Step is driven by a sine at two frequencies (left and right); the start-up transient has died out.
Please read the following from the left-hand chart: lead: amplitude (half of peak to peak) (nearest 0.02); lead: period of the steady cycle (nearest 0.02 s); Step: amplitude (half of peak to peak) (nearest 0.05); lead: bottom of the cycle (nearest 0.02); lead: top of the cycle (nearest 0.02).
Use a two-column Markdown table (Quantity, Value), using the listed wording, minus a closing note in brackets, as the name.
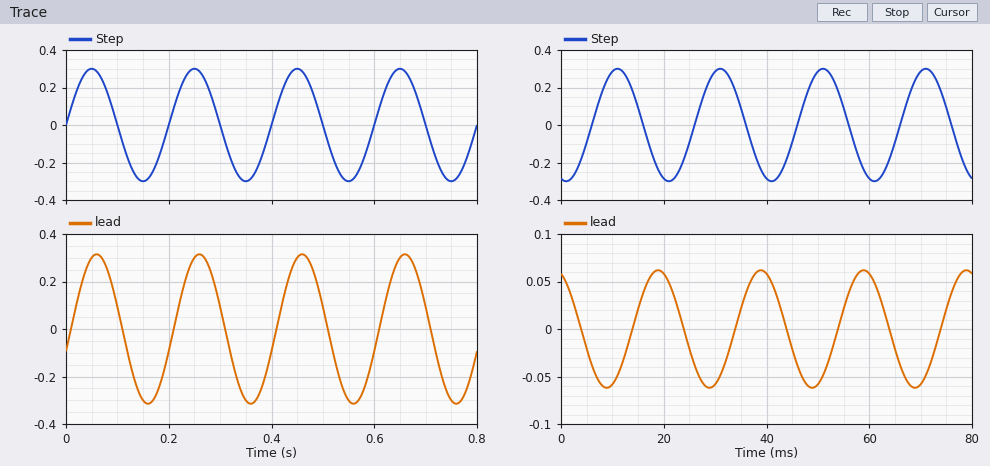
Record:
| Quantity | Value |
|---|---|
| lead: amplitude (half of peak to peak) | 0.32 |
| lead: period of the steady cycle | 0.20 s |
| Step: amplitude (half of peak to peak) | 0.30 |
| lead: bottom of the cycle | -0.32 |
| lead: top of the cycle | 0.32 |
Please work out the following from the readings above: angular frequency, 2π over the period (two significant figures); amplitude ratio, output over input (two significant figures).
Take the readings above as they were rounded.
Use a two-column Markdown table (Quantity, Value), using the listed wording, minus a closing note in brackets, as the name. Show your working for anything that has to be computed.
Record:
| Quantity | Value |
|---|---|
| angular frequency, 2π over the period | 2π / 0.2 = 31 rad/s |
| amplitude ratio, output over input | 0.32 / 0.3 = 1.1 |
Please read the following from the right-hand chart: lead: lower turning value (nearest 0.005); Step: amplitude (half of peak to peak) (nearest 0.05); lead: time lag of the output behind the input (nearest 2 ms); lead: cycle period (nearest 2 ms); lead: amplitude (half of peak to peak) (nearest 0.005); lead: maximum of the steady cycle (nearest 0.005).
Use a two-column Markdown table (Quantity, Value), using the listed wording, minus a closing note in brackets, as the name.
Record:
| Quantity | Value |
|---|---|
| lead: lower turning value | -0.060 |
| Step: amplitude (half of peak to peak) | 0.30 |
| lead: time lag of the output behind the input | 8 ms |
| lead: cycle period | 20 ms |
| lead: amplitude (half of peak to peak) | 0.060 |
| lead: maximum of the steady cycle | 0.060 |
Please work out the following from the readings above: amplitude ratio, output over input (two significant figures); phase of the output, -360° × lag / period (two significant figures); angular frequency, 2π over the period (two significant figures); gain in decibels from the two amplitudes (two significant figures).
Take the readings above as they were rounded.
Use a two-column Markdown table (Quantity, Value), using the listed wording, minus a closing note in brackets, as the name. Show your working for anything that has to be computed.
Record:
| Quantity | Value |
|---|---|
| amplitude ratio, output over input | 0.06 / 0.3 = 0.20 |
| phase of the output, -360° × lag / period | -360 × 8 / 20 = -140° |
| angular frequency, 2π over the period | 2π / 20 = 0.31 rad/ms |
| gain in decibels from the two amplitudes | 20 log10(0.06 / 0.3) = -14 dB |
